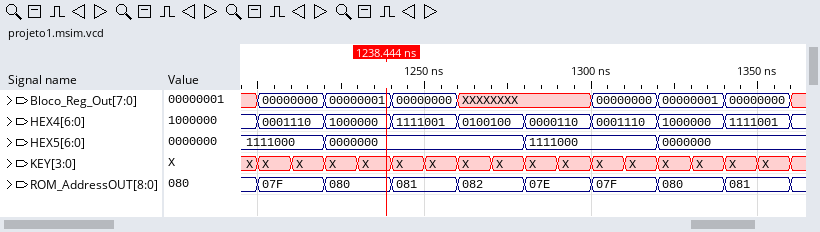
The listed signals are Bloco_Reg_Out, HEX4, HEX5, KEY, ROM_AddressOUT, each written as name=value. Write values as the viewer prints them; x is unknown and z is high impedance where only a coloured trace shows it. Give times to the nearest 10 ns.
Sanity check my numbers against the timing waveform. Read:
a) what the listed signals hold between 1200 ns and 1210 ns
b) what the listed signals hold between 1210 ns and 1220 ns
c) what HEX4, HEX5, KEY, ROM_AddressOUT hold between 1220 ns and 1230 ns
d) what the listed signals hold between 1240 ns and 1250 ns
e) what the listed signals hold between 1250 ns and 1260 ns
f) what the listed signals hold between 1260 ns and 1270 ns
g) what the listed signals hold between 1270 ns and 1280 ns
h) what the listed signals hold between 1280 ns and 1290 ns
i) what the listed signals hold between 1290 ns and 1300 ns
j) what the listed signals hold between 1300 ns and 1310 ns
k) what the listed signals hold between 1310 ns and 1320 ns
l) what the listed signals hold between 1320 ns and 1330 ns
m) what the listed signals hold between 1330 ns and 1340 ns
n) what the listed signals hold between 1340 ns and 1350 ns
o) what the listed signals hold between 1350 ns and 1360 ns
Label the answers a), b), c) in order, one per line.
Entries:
a) Bloco_Reg_Out=00000000, HEX4=0001110, HEX5=1111000, KEY=X, ROM_AddressOUT=07F
b) Bloco_Reg_Out=00000000, HEX4=0001110, HEX5=1111000, KEY=X, ROM_AddressOUT=07F
c) HEX4=1000000, HEX5=0000000, KEY=X, ROM_AddressOUT=080
d) Bloco_Reg_Out=00000000, HEX4=1111001, HEX5=0000000, KEY=X, ROM_AddressOUT=081
e) Bloco_Reg_Out=00000000, HEX4=1111001, HEX5=0000000, KEY=X, ROM_AddressOUT=081
f) Bloco_Reg_Out=XXXXXXXX, HEX4=0100100, HEX5=0000000, KEY=X, ROM_AddressOUT=082
g) Bloco_Reg_Out=XXXXXXXX, HEX4=0100100, HEX5=0000000, KEY=X, ROM_AddressOUT=082
h) Bloco_Reg_Out=XXXXXXXX, HEX4=0000110, HEX5=1111000, KEY=X, ROM_AddressOUT=07E
i) Bloco_Reg_Out=XXXXXXXX, HEX4=0000110, HEX5=1111000, KEY=X, ROM_AddressOUT=07E
j) Bloco_Reg_Out=00000000, HEX4=0001110, HEX5=1111000, KEY=X, ROM_AddressOUT=07F
k) Bloco_Reg_Out=00000000, HEX4=0001110, HEX5=1111000, KEY=X, ROM_AddressOUT=07F
l) Bloco_Reg_Out=00000001, HEX4=1000000, HEX5=0000000, KEY=X, ROM_AddressOUT=080
m) Bloco_Reg_Out=00000001, HEX4=1000000, HEX5=0000000, KEY=X, ROM_AddressOUT=080
n) Bloco_Reg_Out=00000000, HEX4=1111001, HEX5=0000000, KEY=X, ROM_AddressOUT=081
o) Bloco_Reg_Out=00000000, HEX4=1111001, HEX5=0000000, KEY=X, ROM_AddressOUT=081
